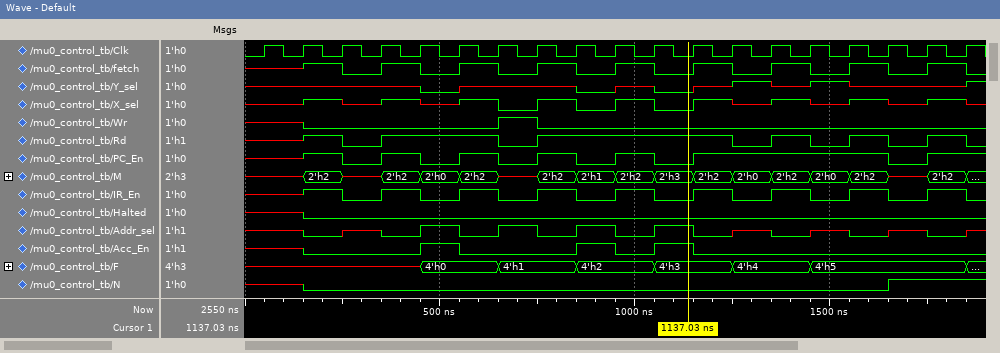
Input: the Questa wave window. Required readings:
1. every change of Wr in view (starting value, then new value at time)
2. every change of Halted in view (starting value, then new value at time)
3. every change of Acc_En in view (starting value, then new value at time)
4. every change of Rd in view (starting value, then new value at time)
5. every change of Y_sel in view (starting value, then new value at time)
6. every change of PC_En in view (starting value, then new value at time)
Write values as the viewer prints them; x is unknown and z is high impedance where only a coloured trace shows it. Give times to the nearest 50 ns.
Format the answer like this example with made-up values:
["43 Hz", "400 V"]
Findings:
["x, 0 at 150 ns, 1 at 650 ns, 0 at 750 ns", "x, 0 at 150 ns", "x, 0 at 150 ns, 1 at 450 ns, 0 at 550 ns, 1 at 850 ns, 0 at 950 ns, 1 at 1050 ns, 0 at 1150 ns", "x, 1 at 150 ns, 0 at 250 ns, 1 at 350 ns, 0 at 650 ns, 1 at 750 ns, 0 at 1250 ns, 1 at 1350 ns, 0 at 1450 ns, 1 at 1550 ns, 0 at 1650 ns, 1 at 1750 ns, 0 at 1850 ns", "x, 0 at 450 ns, x at 550 ns, 0 at 850 ns, x at 950 ns, 0 at 1050 ns, x at 1150 ns, 1 at 1250 ns, x at 1350 ns, 1 at 1450 ns, x at 1550 ns, 1 at 1850 ns", "x, 1 at 150 ns, 0 at 250 ns, 1 at 350 ns, 0 at 450 ns, 1 at 550 ns, 0 at 650 ns, 1 at 750 ns, 0 at 850 ns, 1 at 950 ns, 0 at 1050 ns, 1 at 1150 ns, 0 at 1650 ns, 1 at 1750 ns"]
